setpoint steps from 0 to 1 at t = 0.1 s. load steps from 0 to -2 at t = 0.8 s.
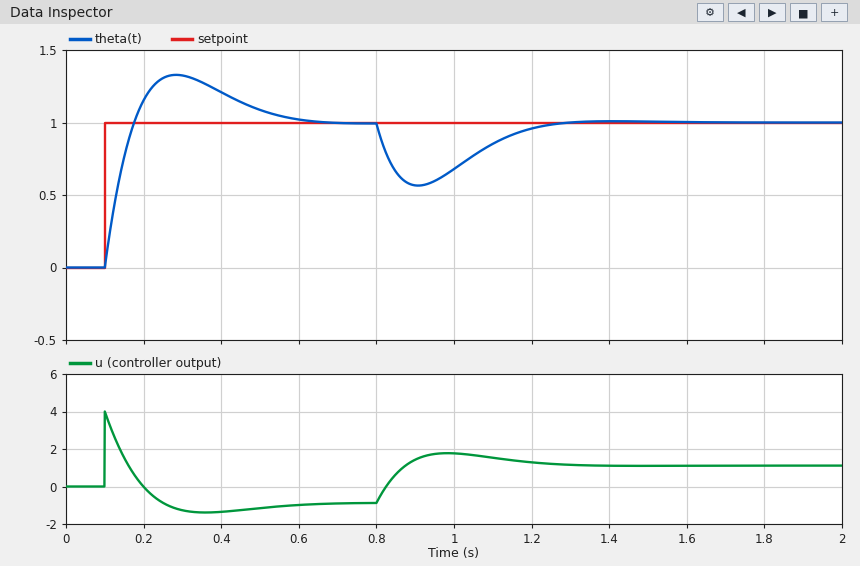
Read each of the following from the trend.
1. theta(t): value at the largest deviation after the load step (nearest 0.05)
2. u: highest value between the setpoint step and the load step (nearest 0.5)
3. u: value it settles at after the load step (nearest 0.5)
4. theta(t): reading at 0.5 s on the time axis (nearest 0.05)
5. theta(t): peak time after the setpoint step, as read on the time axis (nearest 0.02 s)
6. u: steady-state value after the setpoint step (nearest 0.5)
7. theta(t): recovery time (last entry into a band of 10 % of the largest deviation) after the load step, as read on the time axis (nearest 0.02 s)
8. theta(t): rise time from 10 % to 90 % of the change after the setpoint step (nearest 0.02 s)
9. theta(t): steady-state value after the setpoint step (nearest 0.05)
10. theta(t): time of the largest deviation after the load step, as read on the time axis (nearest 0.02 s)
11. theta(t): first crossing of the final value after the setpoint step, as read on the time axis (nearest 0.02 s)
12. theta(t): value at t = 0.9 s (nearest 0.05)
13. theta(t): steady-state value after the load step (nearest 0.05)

0.55
4.0
1.0
1.10
0.28 s
-1.0
1.20 s
0.06 s
1.00
0.90 s
0.18 s
0.55
1.00
